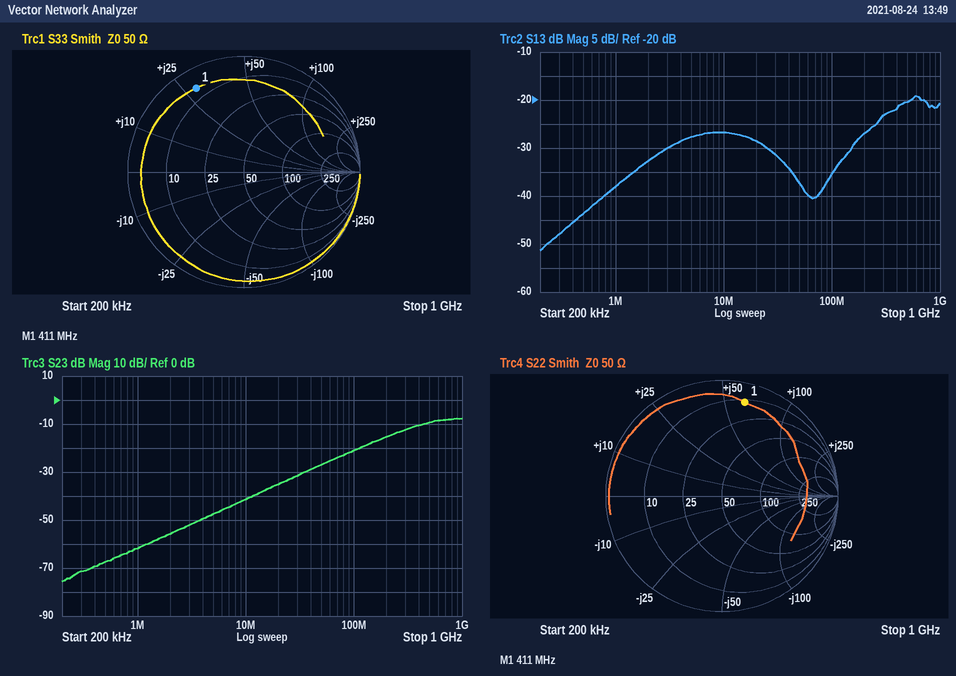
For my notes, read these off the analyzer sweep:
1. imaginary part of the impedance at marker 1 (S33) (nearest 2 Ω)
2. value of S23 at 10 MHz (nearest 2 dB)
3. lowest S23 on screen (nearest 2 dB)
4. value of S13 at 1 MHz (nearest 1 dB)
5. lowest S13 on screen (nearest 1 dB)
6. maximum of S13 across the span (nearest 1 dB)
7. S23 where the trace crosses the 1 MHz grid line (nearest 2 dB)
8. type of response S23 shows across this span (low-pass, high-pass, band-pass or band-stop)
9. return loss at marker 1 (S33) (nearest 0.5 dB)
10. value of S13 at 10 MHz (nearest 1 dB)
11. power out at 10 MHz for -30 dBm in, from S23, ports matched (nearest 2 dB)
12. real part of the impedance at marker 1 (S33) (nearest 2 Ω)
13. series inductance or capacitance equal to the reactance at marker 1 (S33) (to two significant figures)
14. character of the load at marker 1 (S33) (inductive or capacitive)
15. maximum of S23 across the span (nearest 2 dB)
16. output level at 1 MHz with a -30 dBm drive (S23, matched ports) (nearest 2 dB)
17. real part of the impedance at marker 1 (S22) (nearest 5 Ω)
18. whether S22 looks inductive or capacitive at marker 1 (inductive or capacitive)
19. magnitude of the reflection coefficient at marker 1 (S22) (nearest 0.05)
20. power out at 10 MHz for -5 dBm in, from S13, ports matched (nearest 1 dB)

+28 Ω
-42 dB
-76 dB
-38 dB
-51 dB
-19 dB
-62 dB
high-pass
1.5 dB
-27 dB
-72 dBm
6 Ω
11 nH
inductive
-8 dB
-92 dBm
10 Ω
inductive
0.85
-32 dBm
